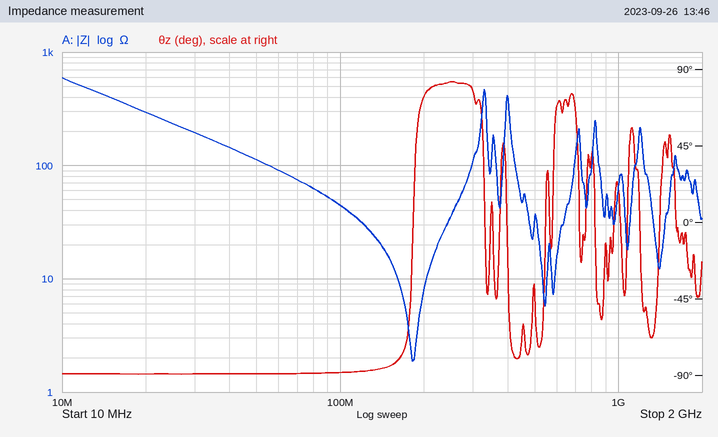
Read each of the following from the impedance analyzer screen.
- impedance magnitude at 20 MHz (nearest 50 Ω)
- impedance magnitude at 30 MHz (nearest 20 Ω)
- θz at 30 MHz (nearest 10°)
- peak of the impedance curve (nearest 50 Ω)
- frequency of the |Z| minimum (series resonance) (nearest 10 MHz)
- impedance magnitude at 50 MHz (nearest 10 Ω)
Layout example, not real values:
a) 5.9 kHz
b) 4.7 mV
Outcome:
a) 300 Ω
b) 200 Ω
c) -90°
d) 600 Ω
e) 180 MHz
f) 110 Ω
